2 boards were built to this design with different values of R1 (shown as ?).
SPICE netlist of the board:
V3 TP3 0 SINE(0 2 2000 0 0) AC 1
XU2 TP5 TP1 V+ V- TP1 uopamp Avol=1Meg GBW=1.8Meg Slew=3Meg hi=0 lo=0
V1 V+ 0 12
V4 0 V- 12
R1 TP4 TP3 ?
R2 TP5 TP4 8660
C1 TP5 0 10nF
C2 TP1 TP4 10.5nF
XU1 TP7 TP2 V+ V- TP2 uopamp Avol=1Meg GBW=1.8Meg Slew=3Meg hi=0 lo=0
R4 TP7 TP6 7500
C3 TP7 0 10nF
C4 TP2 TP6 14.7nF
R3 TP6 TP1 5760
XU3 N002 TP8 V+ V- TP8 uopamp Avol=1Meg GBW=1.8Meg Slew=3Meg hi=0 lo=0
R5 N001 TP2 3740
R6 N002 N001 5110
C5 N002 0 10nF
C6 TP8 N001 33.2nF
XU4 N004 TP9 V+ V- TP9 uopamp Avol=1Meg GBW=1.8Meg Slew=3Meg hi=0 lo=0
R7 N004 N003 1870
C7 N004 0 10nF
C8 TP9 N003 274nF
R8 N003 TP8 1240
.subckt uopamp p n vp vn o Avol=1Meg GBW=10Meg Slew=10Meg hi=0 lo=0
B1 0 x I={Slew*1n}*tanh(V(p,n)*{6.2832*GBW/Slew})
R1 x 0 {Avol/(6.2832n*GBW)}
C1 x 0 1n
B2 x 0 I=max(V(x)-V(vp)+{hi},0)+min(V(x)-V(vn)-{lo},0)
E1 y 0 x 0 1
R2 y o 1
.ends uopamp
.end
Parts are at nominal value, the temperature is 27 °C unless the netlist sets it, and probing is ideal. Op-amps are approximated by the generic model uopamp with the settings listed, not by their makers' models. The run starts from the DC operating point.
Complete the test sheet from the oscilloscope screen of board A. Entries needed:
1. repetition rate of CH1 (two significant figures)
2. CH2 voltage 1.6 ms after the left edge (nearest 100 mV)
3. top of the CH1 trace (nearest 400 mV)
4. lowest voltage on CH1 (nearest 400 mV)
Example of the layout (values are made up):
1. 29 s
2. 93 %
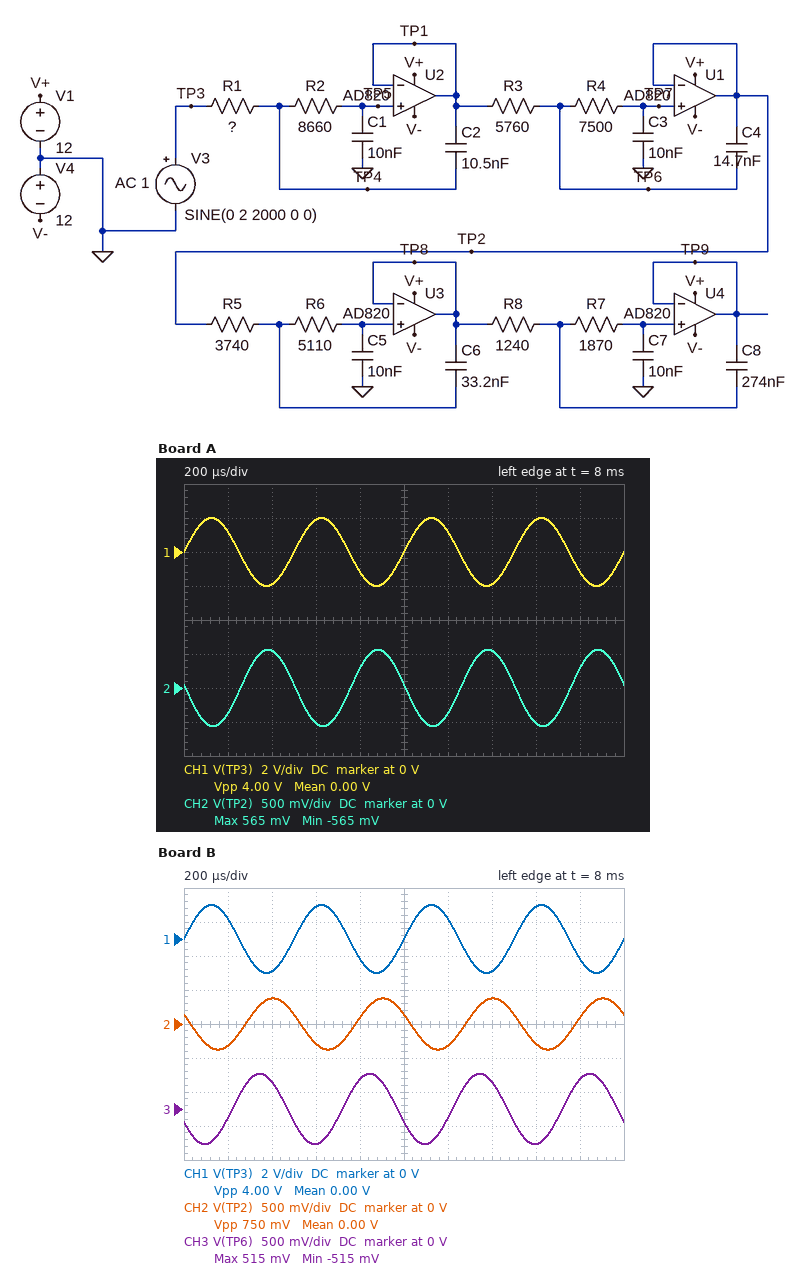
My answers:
1. 2.0 kHz
2. -500 mV
3. 2.0 V
4. -2.0 V
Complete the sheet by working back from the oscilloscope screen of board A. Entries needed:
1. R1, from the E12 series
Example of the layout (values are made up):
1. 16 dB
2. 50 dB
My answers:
1. 8.2 kΩ
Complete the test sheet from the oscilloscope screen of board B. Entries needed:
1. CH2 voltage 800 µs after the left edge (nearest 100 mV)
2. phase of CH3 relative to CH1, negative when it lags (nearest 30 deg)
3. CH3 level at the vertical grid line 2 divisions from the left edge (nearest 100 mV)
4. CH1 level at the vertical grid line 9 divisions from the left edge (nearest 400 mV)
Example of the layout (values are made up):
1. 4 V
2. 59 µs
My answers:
1. 100 mV
2. -150 deg
3. 400 mV
4. -1.2 V
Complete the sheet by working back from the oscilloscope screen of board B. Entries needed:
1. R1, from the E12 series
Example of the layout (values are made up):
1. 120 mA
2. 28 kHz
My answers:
1. 15 kΩ
